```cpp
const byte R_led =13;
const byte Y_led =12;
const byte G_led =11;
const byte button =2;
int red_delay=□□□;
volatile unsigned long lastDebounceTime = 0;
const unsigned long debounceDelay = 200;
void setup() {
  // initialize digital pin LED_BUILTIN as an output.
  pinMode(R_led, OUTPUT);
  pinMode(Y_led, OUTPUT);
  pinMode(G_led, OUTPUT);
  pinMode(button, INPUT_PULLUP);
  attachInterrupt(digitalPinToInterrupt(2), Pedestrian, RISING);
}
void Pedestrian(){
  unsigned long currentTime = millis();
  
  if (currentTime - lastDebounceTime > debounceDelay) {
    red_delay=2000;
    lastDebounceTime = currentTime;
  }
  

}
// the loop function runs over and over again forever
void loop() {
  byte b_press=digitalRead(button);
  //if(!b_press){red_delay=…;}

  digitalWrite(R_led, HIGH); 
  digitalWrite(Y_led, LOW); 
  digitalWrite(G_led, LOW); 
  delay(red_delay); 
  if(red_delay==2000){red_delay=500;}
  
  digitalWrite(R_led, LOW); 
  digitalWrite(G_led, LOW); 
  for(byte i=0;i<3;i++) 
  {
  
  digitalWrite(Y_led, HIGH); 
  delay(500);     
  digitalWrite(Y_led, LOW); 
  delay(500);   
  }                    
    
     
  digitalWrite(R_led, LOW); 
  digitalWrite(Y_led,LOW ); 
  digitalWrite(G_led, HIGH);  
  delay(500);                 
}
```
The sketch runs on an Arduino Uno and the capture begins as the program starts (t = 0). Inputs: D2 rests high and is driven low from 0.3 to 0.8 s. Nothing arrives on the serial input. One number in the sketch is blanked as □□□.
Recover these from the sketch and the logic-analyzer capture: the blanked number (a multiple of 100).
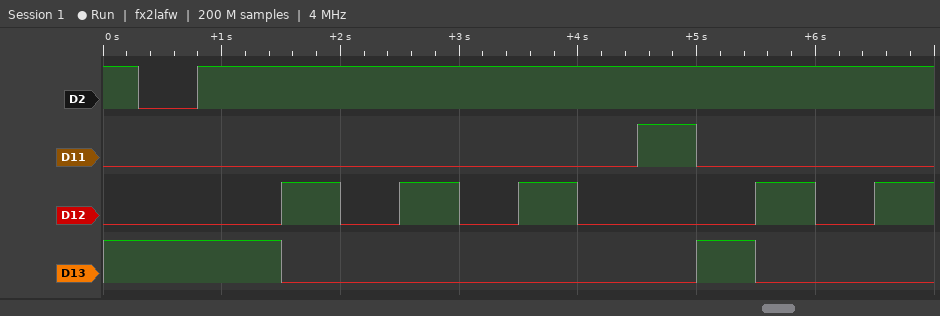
1500
